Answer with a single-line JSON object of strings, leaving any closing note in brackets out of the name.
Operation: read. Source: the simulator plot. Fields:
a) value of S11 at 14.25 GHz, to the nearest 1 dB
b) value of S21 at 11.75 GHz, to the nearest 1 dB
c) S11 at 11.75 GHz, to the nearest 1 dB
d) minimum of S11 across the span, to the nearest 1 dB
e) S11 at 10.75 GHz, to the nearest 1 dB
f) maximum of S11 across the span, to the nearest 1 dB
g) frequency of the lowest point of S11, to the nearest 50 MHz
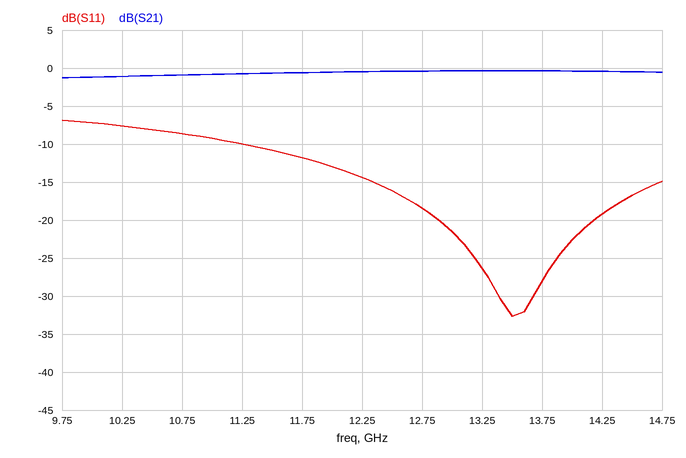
{"value of S11 at 14.25 GHz, to the nearest 1 dB": "-19 dB", "value of S21 at 11.75 GHz, to the nearest 1 dB": "-1 dB", "S11 at 11.75 GHz, to the nearest 1 dB": "-12 dB", "minimum of S11 across the span, to the nearest 1 dB": "-33 dB", "S11 at 10.75 GHz, to the nearest 1 dB": "-9 dB", "maximum of S11 across the span, to the nearest 1 dB": "-7 dB", "frequency of the lowest point of S11, to the nearest 50 MHz": "13.50 GHz"}
